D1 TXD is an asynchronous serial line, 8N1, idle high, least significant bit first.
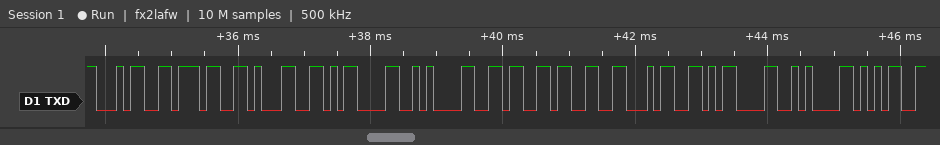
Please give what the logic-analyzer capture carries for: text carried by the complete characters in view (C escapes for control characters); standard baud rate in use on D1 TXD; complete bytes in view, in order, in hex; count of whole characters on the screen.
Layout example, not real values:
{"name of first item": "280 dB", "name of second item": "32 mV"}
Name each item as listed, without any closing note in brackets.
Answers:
{"text carried by the complete characters in view": "\"471\\r\\n634\\r\\n5\"", "standard baud rate in use on D1 TXD": "9600 baud", "complete bytes in view, in order, in hex": "0x34 0x37 0x31 0x0D 0x0A 0x36 0x33 0x34 0x0D 0x0A 0x35", "count of whole characters on the screen": "11"}
